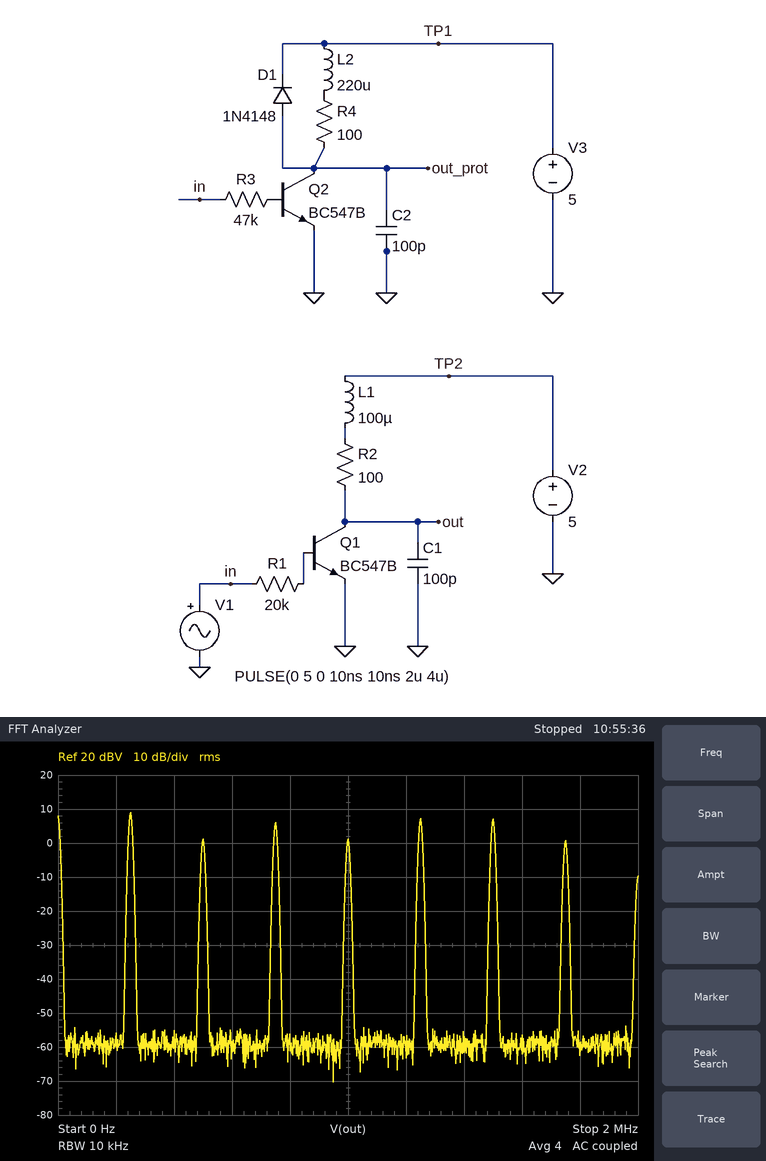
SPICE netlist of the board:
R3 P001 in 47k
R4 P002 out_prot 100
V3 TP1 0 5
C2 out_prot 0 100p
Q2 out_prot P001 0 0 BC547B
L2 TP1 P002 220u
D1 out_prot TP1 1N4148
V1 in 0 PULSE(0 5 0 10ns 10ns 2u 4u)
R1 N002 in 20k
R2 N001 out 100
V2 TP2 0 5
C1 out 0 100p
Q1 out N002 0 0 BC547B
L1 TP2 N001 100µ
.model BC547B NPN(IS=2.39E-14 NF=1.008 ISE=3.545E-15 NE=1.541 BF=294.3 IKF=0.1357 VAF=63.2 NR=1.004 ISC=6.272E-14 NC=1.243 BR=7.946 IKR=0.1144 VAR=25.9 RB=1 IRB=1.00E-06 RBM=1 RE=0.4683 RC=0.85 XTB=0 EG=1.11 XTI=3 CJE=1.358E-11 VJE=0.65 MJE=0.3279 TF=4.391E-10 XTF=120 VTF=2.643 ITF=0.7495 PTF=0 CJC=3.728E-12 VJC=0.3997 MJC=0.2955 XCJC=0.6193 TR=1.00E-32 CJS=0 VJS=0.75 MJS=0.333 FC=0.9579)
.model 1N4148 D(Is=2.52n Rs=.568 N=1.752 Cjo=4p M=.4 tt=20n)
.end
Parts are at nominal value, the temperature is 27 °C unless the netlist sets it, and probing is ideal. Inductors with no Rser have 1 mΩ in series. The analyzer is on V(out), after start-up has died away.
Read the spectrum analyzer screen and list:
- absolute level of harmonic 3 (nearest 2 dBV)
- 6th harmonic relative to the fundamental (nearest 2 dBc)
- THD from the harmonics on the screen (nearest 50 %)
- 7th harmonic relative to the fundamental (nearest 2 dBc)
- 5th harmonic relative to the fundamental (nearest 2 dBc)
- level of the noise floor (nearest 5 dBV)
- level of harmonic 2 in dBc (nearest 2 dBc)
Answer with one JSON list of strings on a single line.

["6 dBV", "-2 dBc", "150 %", "-8 dBc", "-2 dBc", "-60 dBV", "-8 dBc"]
